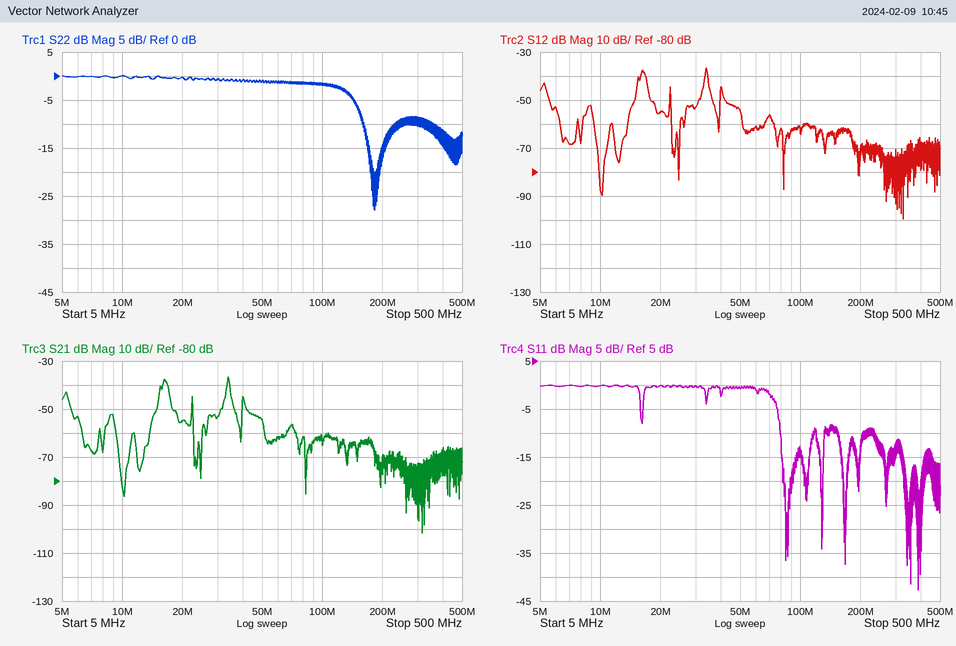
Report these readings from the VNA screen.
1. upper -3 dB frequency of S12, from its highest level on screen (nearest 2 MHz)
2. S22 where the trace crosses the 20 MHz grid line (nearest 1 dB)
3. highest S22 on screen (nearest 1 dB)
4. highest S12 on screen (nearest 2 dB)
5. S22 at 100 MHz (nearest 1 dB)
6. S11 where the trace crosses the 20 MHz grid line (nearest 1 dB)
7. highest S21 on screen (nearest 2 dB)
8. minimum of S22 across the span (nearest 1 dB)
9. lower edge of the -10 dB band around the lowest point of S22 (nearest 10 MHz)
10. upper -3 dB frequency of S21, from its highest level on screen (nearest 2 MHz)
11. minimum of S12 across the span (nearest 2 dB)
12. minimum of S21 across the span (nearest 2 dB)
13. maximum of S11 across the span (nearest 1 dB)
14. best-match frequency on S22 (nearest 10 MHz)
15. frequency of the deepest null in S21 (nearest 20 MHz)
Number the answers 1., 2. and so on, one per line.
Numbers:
1. 34 MHz
2. 0 dB
3. 0 dB
4. -36 dB
5. -2 dB
6. 0 dB
7. -36 dB
8. -28 dB
9. 160 MHz
10. 34 MHz
11. -100 dB
12. -102 dB
13. 0 dB
14. 180 MHz
15. 320 MHz
